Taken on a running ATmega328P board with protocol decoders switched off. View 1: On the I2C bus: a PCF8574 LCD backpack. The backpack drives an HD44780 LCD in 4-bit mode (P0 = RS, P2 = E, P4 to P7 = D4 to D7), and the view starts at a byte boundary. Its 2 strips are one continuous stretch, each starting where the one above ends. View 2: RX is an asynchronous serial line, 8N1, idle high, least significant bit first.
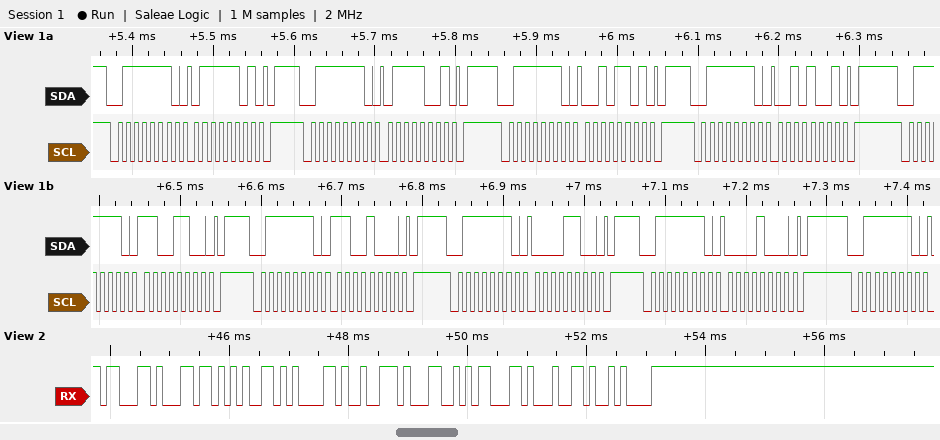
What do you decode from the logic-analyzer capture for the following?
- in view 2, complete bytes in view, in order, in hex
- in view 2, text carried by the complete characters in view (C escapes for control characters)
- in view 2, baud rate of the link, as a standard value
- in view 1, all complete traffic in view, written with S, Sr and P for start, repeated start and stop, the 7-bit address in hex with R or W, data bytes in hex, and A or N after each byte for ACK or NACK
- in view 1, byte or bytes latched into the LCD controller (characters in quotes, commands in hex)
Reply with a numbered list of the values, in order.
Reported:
1. 63 6C 65 61 72 4C 63 64 0A
2. "clearLcd\n"
3. 9600 baud
4. S 3FW A 7D A P S 3FW A 79 A P S 3FW A 2D A P S 3FW A 29 A P S 3FW A CC A P S 3FW A C8 A P S 3FW A 0C A P S 3FW A 08 A P S 3FW A
5. 'r' 0xC0
